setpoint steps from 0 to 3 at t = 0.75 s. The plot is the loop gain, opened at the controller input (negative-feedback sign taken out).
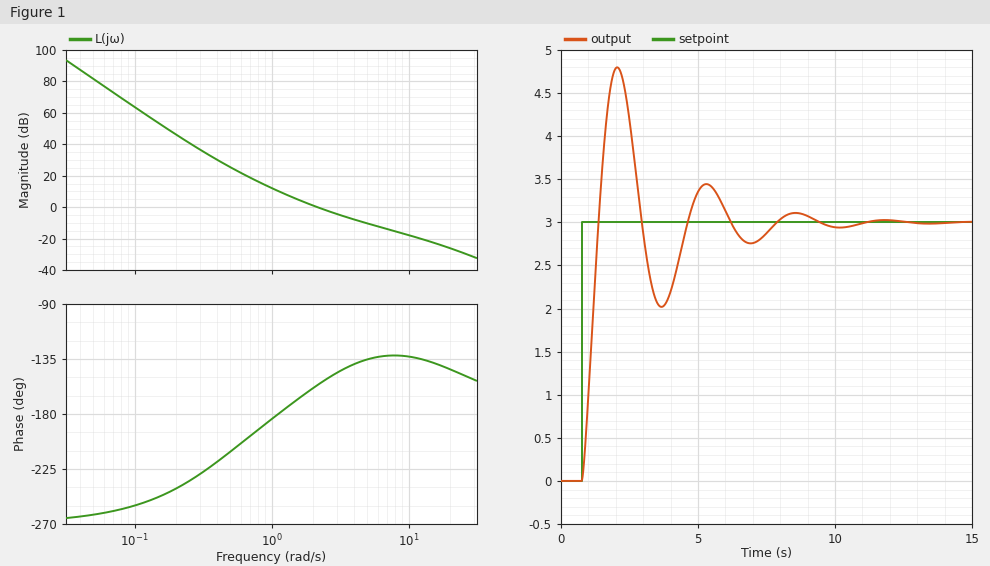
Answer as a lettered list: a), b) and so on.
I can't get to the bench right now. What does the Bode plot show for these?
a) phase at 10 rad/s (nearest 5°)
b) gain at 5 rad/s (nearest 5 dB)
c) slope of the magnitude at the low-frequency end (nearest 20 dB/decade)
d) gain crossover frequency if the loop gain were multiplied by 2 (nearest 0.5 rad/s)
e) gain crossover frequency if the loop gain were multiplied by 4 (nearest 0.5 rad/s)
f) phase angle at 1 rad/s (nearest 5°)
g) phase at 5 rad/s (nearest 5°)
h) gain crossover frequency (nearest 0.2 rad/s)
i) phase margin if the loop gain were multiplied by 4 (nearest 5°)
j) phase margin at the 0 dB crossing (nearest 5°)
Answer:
a) -135°
b) -10 dB
c) -60 dB/decade
d) 3.5 rad/s
e) 6.0 rad/s
f) -185°
g) -135°
h) 2.2 rad/s
i) 45°
j) 25°
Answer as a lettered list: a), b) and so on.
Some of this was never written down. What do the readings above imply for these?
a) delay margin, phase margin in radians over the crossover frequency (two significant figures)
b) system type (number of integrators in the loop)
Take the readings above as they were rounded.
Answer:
a) 0.20 s
b) 3
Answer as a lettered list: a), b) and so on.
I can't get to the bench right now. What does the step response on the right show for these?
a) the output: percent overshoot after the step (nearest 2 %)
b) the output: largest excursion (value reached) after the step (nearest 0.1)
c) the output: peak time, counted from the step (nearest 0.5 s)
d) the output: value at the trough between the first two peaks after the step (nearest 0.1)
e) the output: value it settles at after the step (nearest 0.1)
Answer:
a) 60 %
b) 4.8
c) 1.5 s
d) 2.0
e) 3.0
